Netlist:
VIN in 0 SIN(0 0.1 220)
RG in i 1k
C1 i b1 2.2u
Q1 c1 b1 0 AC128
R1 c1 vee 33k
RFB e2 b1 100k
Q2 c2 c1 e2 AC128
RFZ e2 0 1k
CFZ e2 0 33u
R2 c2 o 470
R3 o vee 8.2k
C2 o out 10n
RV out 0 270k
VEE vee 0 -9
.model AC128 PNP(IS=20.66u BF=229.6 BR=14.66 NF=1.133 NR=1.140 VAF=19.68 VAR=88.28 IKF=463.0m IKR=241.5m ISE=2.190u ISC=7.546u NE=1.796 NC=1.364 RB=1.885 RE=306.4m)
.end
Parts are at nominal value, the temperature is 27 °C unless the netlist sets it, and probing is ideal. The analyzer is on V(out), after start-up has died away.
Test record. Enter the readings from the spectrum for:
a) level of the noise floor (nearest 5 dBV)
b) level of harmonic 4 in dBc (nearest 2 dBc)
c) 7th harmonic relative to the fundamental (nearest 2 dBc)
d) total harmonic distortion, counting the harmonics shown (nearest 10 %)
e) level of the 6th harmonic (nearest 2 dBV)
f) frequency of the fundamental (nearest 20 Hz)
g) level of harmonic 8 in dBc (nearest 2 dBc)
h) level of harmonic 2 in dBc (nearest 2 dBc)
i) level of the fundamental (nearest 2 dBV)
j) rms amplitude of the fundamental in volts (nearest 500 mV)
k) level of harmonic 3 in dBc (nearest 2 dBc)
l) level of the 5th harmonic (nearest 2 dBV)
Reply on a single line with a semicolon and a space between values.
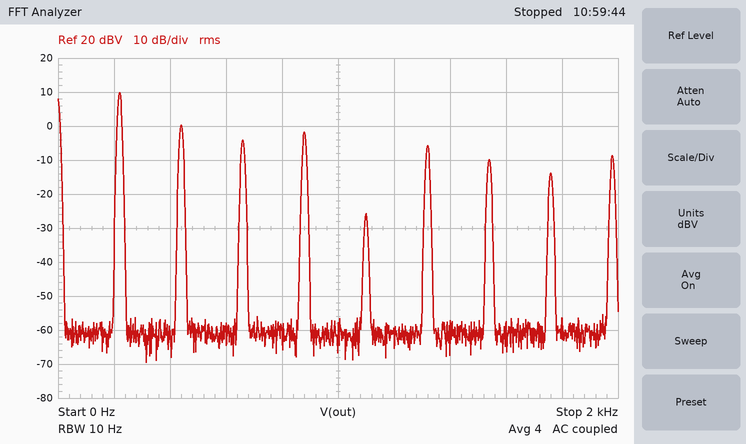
-60 dBV; -12 dBc; -20 dBc; 50 %; -6 dBV; 220 Hz; -24 dBc; -10 dBc; 10 dBV; 3.0 V; -14 dBc; -26 dBV
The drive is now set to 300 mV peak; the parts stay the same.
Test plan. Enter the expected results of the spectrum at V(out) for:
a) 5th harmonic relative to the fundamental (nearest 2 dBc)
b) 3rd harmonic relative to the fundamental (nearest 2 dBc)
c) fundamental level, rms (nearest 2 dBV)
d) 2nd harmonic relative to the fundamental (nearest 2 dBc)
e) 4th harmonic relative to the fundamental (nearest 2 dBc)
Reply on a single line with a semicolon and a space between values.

-12 dBc; -16 dBc; 8 dBV; -4 dBc; -16 dBc
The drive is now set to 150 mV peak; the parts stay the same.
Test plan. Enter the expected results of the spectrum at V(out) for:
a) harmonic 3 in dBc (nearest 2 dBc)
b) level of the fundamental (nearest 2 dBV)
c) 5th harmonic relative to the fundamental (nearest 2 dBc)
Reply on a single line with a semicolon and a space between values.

-22 dBc; 10 dBV; -16 dBc
